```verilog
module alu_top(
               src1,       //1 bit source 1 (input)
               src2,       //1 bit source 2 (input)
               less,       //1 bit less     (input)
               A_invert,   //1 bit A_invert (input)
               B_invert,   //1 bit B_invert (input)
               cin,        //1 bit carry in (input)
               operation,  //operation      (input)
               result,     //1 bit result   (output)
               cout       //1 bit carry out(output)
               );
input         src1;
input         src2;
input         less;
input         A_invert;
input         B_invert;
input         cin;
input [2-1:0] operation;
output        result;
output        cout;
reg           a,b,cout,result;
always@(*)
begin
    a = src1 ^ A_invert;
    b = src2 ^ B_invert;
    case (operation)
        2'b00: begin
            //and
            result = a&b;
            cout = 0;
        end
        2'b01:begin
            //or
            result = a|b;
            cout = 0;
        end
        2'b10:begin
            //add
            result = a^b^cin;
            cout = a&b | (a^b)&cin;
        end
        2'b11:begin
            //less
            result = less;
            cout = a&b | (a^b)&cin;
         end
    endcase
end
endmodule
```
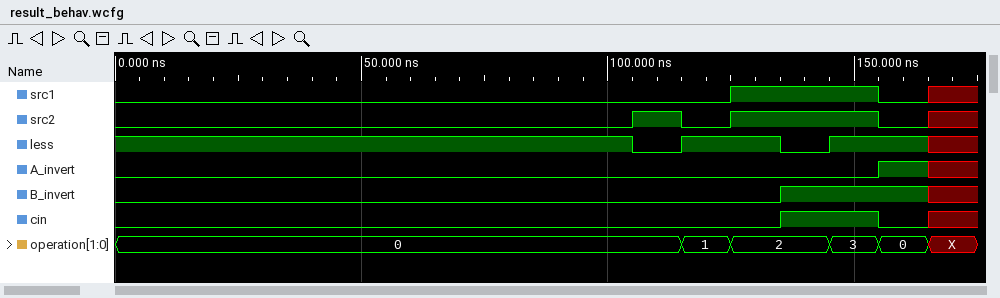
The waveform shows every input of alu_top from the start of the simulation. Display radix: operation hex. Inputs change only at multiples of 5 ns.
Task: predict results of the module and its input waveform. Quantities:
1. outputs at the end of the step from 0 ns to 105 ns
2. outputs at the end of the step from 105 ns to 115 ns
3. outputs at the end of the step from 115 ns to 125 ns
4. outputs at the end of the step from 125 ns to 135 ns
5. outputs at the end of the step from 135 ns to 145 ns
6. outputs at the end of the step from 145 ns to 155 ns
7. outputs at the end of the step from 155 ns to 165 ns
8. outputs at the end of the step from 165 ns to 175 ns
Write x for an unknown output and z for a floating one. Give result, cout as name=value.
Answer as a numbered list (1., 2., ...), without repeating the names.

1. result=0, cout=0
2. result=0, cout=0
3. result=0, cout=0
4. result=0, cout=1
5. result=0, cout=1
6. result=1, cout=1
7. result=1, cout=0
8. result=1, cout=0
